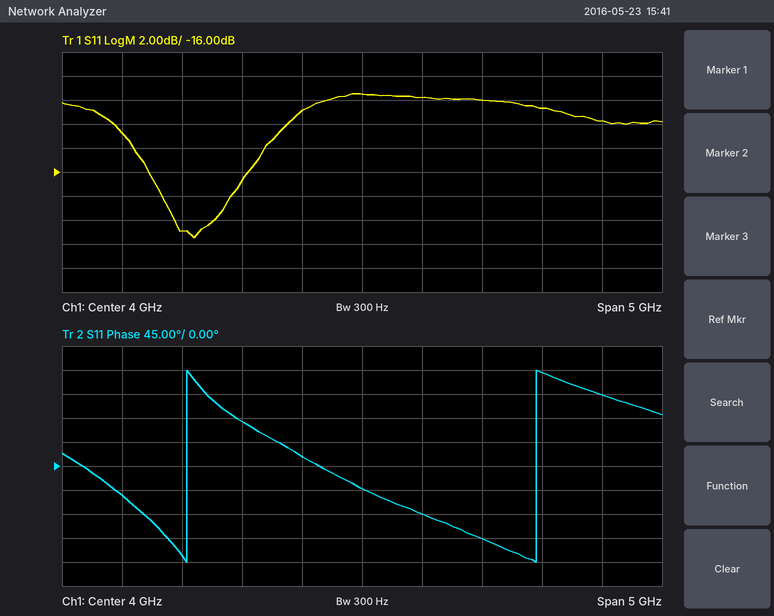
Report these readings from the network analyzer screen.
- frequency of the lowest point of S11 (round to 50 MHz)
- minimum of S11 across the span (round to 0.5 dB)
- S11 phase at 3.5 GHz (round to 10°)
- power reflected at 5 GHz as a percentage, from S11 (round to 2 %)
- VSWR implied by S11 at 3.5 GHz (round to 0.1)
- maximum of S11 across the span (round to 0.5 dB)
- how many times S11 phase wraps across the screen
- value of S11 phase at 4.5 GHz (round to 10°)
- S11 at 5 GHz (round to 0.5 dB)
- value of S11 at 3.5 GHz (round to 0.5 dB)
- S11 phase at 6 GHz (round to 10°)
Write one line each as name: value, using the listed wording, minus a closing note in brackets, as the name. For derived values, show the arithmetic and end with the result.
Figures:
frequency of the lowest point of S11: 2.60 GHz
minimum of S11 across the span: -21.5 dB
S11 phase at 3.5 GHz: 20°
power reflected at 5 GHz as a percentage, from S11: 10^(-10/10) ≈ 10 %
VSWR implied by S11 at 3.5 GHz: |Γ| = 10^(-11/20) = 0.2818; VSWR = (1 + 0.2818)/(1 − 0.2818) ≈ 1.8
maximum of S11 across the span: -9.5 dB
how many times S11 phase wraps across the screen: 2
value of S11 phase at 4.5 GHz: -90°
S11 at 5 GHz: -10.0 dB
value of S11 at 3.5 GHz: -11.0 dB
S11 phase at 6 GHz: 130°
